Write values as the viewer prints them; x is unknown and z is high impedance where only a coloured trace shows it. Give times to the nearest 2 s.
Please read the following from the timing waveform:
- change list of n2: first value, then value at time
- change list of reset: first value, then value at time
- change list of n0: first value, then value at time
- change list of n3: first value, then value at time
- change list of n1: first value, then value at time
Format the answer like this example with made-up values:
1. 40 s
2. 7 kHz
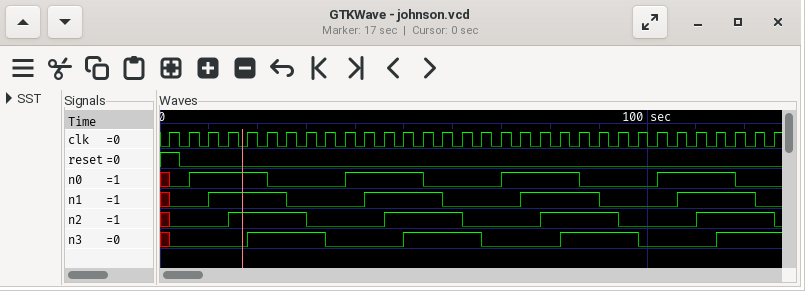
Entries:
1. x, 0 at 2 s, 1 at 14 s, 0 at 30 s, 1 at 46 s, 0 at 62 s, 1 at 78 s, 0 at 94 s, 1 at 110 s, 0 at 126 s
2. 1, 0 at 4 s
3. x, 0 at 2 s, 1 at 6 s, 0 at 22 s, 1 at 38 s, 0 at 54 s, 1 at 70 s, 0 at 86 s, 1 at 102 s, 0 at 118 s
4. x, 0 at 2 s, 1 at 18 s, 0 at 34 s, 1 at 50 s, 0 at 66 s, 1 at 82 s, 0 at 98 s, 1 at 114 s
5. x, 0 at 2 s, 1 at 10 s, 0 at 26 s, 1 at 42 s, 0 at 58 s, 1 at 74 s, 0 at 90 s, 1 at 106 s, 0 at 122 s
